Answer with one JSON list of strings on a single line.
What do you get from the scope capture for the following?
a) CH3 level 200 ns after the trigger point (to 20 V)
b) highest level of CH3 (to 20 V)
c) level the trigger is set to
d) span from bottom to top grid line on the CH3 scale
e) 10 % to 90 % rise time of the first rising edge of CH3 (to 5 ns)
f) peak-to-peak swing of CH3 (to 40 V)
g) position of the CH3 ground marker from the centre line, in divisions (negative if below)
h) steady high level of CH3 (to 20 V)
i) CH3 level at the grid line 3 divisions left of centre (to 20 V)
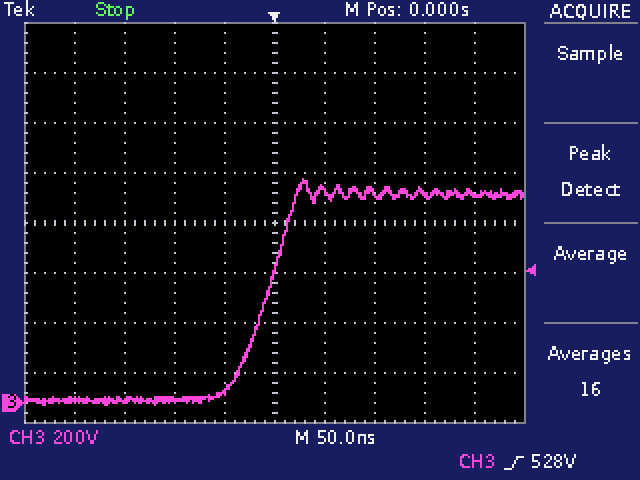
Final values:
["840 V", "900 V", "528 V", "1.6 kV", "55 ns", "920 V", "-3.6 div", "840 V", "20 V"]
